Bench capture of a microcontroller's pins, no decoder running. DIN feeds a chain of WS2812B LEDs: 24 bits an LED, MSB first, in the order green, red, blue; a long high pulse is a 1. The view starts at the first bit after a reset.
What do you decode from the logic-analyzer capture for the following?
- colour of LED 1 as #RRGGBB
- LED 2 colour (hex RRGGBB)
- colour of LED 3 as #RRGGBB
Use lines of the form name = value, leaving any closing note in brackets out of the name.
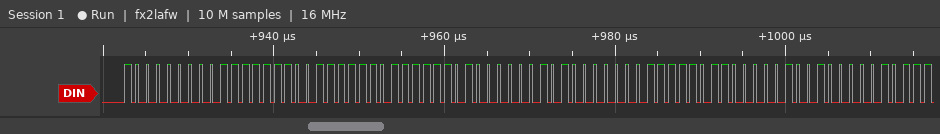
colour of LED 1 as #RRGGBB = #7F803F
LED 2 colour = #817E40
colour of LED 3 as #RRGGBB = #827D41
